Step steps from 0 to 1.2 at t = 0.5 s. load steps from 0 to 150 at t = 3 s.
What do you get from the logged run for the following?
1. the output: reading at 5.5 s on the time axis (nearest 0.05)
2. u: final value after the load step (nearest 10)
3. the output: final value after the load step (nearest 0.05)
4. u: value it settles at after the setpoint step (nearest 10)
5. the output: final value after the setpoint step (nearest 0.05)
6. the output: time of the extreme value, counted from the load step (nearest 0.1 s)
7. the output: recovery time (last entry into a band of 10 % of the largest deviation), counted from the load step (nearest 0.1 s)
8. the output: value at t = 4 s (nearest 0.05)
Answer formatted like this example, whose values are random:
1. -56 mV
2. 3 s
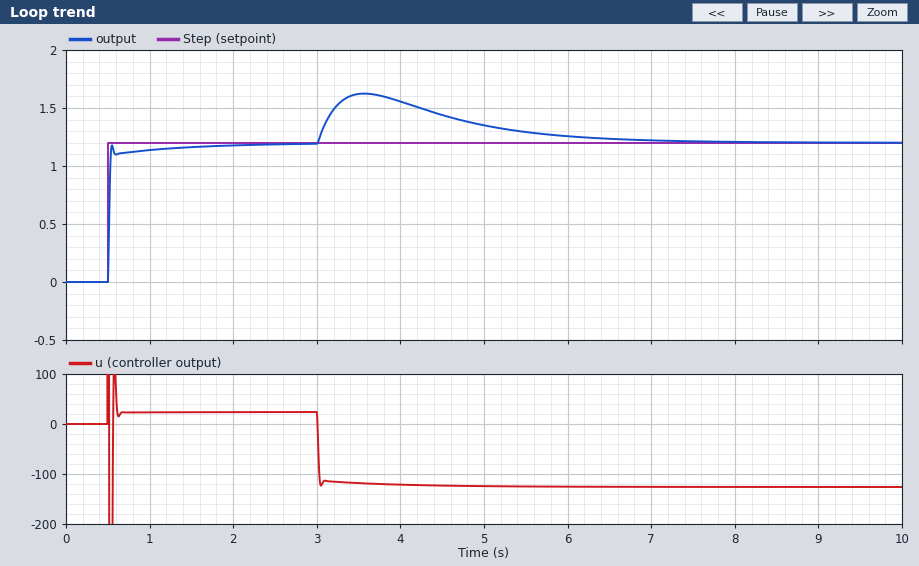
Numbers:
1. 1.30
2. -130
3. 1.20
4. 20
5. 1.20
6. 0.6 s
7. 3.3 s
8. 1.55
